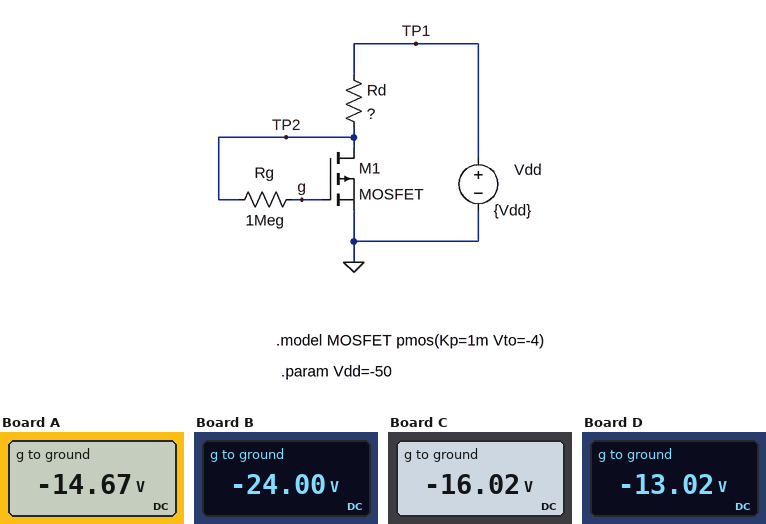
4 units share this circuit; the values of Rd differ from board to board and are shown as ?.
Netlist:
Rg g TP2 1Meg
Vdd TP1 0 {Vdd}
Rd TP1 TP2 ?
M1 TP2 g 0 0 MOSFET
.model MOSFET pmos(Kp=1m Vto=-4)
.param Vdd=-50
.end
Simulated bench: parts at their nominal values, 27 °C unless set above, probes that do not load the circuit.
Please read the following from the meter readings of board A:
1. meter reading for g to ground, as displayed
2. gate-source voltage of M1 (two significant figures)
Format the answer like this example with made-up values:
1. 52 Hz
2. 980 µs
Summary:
1. -14.67 V
2. -15 V
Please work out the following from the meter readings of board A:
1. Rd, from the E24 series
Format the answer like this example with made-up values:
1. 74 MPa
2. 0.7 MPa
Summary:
1. 620 Ω
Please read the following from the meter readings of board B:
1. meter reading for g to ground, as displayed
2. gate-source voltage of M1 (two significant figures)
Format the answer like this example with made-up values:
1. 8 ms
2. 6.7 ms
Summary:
1. -24.00 V
2. -24 V
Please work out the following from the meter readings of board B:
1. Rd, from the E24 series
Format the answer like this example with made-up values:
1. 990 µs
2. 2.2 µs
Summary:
1. 130 Ω
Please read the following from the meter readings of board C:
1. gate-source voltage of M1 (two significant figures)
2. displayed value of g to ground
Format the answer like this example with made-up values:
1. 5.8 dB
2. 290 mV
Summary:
1. -16 V
2. -16.02 V
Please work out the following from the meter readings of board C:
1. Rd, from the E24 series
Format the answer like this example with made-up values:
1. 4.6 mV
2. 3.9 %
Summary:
1. 470 Ω
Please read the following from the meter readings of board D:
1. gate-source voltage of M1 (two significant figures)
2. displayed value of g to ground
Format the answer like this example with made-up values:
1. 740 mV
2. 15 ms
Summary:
1. -13 V
2. -13.02 V
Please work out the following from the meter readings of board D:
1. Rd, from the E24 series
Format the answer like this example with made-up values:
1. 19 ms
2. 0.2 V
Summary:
1. 910 Ω
